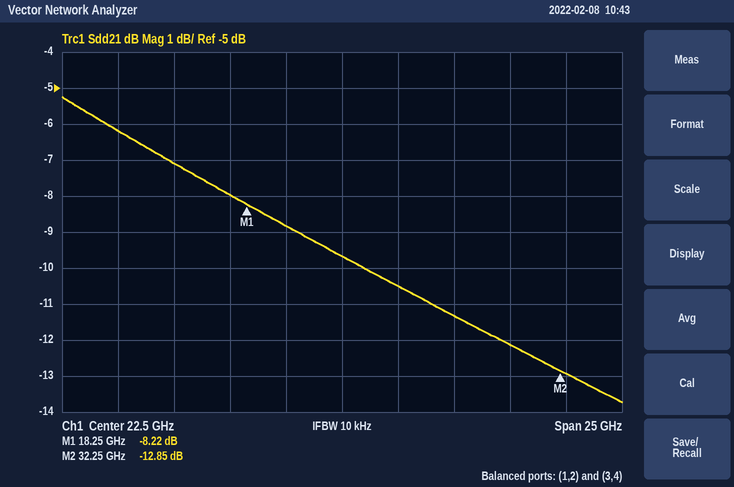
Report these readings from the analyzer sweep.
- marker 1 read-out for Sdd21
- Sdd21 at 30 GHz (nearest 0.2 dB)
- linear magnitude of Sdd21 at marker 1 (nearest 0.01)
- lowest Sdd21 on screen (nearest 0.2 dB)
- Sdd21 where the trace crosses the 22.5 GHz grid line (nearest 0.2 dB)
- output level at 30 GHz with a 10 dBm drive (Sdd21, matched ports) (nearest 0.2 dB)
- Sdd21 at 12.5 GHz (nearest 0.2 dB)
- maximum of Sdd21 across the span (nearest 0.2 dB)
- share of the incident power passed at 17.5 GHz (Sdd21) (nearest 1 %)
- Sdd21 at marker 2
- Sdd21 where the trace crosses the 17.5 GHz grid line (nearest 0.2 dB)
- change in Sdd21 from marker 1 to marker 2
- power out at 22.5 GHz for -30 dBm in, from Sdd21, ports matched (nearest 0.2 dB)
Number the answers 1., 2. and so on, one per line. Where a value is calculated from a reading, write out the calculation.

1. -8.22 dB
2. -12.2 dB
3. 10^(-8.22/20) ≈ 0.39
4. -13.8 dB
5. -9.6 dB
6. 10 dBm + (-12.2 dB) = -2.2 dBm
7. -6.2 dB
8. -5.2 dB
9. 10^(-8/10) ≈ 16 %
10. -12.85 dB
11. -8.0 dB
12. -12.85 − (-8.22) = -4.63 dB
13. -30 dBm + (-9.6 dB) = -39.6 dBm
